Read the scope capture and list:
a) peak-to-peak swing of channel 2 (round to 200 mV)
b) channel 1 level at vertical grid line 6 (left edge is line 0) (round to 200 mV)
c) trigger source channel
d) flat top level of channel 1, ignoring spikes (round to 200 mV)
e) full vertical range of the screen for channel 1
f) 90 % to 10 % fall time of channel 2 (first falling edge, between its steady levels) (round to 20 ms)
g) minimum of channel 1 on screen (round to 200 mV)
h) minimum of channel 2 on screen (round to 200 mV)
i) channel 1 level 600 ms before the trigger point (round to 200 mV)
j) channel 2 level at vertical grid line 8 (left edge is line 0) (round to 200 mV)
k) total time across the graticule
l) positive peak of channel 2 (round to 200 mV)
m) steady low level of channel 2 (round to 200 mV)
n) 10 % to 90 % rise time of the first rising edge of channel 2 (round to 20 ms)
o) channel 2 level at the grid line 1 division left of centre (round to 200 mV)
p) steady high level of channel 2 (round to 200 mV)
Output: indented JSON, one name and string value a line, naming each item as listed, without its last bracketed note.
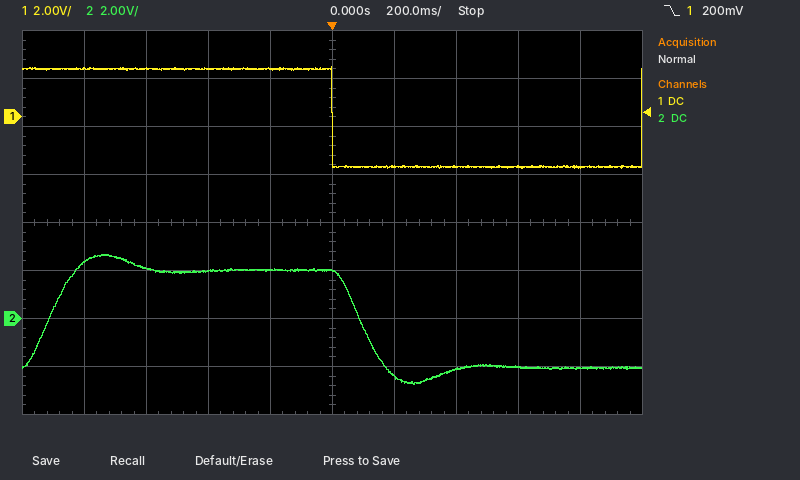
{
  "peak-to-peak swing of channel 2": "5.4 V",
  "channel 1 level at vertical grid line 6 (left edge is line 0)": "-2.0 V",
  "trigger source channel": "channel 1",
  "flat top level of channel 1, ignoring spikes": "2.0 V",
  "full vertical range of the screen for channel 1": "16 V",
  "90 % to 10 % fall time of channel 2 (first falling edge, between its steady levels)": "120 ms",
  "minimum of channel 1 on screen": "-2.2 V",
  "minimum of channel 2 on screen": "-2.8 V",
  "channel 1 level 600 ms before the trigger point": "2.0 V",
  "channel 2 level at vertical grid line 8 (left edge is line 0)": "-2.0 V",
  "total time across the graticule": "2 s",
  "positive peak of channel 2": "2.6 V",
  "steady low level of channel 2": "-2.0 V",
  "10 % to 90 % rise time of the first rising edge of channel 2": "120 ms",
  "channel 2 level at the grid line 1 division left of centre": "2.0 V",
  "steady high level of channel 2": "2.0 V"
}
